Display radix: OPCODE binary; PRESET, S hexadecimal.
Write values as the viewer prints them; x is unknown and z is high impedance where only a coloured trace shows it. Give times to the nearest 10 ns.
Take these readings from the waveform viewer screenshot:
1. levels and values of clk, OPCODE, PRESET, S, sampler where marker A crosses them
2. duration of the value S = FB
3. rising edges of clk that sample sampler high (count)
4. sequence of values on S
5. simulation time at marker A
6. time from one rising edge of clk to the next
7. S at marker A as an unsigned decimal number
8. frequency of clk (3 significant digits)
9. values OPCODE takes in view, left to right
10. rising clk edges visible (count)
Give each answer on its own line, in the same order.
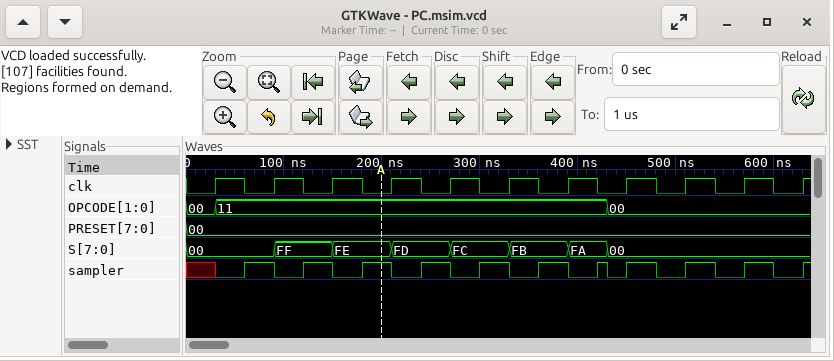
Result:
clk=0, OPCODE=11, PRESET=00, S=FE, sampler=1
60 ns
6
00, FF, FE, FD, FC, FB, FA, 00
200 ns
60 ns
254
16.7 MHz
00, 11, 00
11
